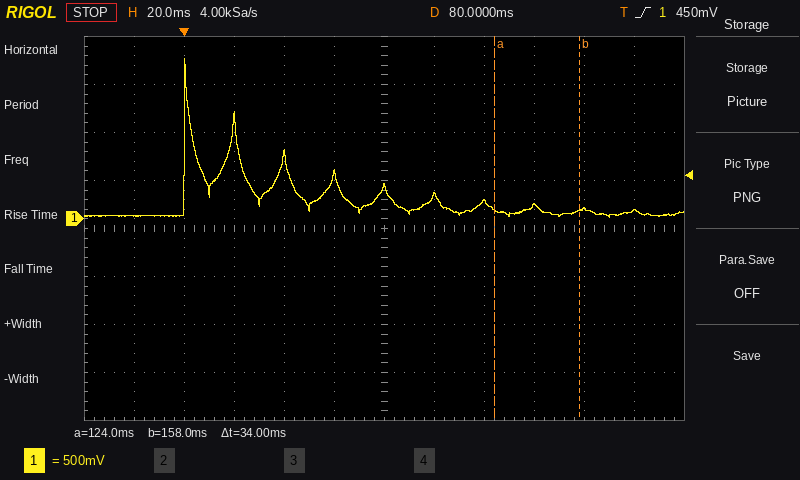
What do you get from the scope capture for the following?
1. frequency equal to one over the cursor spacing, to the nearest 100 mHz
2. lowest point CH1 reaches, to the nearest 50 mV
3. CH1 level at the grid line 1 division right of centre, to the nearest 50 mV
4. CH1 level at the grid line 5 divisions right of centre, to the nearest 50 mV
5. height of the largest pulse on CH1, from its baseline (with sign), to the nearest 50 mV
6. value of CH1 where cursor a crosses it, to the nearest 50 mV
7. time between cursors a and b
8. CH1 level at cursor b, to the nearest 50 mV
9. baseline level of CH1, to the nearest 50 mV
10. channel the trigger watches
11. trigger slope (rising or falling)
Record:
29.4 Hz
0 mV
250 mV
100 mV
+1.60 V
100 mV
34 ms
100 mV
50 mV
CH1
rising
